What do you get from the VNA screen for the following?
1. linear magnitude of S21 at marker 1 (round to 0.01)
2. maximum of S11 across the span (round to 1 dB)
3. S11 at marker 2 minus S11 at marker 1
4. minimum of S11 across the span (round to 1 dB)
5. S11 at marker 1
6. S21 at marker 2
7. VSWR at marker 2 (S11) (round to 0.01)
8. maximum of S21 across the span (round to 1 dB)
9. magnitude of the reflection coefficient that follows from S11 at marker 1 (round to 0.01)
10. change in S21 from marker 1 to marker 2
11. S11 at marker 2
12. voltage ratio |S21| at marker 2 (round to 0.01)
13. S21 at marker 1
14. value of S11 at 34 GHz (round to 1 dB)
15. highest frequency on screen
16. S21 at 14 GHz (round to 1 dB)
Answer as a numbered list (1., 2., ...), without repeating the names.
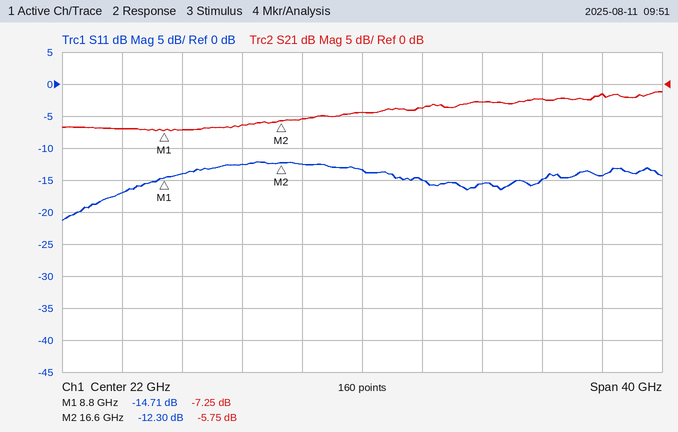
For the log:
1. 0.43
2. -12 dB
3. 2.41 dB
4. -21 dB
5. -14.71 dB
6. -5.75 dB
7. 1.64
8. -1 dB
9. 0.18
10. 1.50 dB
11. -12.30 dB
12. 0.52
13. -7.25 dB
14. -15 dB
15. 42 GHz
16. -6 dB
